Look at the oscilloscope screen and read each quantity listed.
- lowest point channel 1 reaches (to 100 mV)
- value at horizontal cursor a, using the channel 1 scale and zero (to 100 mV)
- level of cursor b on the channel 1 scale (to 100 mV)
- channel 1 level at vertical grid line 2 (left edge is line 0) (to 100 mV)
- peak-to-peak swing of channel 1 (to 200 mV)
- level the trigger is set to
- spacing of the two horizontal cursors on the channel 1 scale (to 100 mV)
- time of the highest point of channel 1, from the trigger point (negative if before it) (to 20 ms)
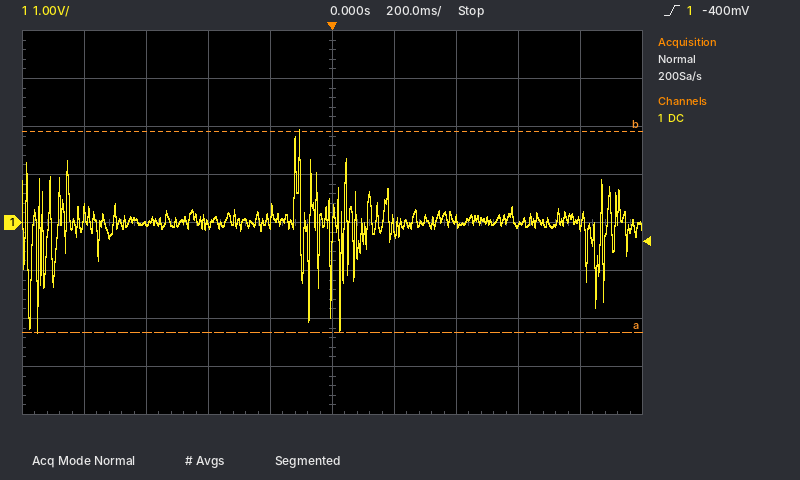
-2.3 V
-2.3 V
1.9 V
0.0 V
4.2 V
-400 mV
4.2 V
-100 ms
